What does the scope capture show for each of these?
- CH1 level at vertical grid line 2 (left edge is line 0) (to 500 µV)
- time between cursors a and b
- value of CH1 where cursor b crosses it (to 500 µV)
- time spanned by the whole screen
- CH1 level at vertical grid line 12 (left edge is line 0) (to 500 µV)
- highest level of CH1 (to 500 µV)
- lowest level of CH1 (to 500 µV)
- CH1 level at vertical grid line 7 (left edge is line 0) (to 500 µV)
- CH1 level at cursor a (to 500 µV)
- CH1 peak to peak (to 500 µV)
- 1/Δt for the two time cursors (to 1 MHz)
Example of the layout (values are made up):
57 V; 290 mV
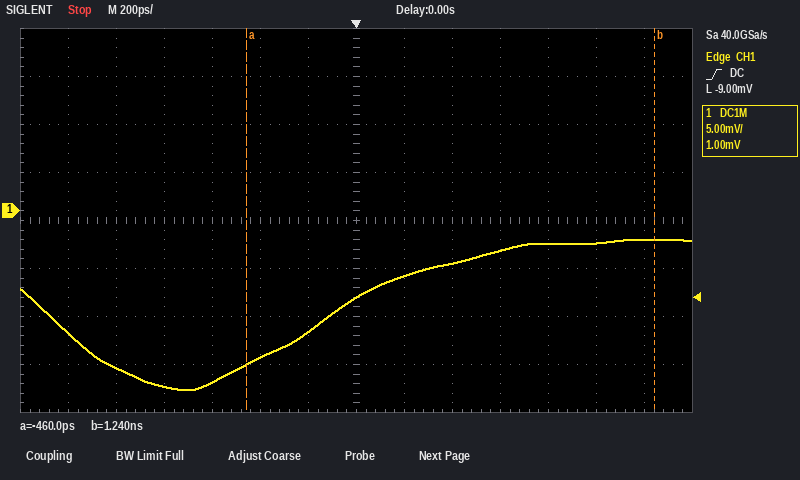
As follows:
-16.5 mV; 1.70 ns; -3.0 mV; 2.8 ns; -3.5 mV; -3.0 mV; -18.5 mV; -9.0 mV; -16.0 mV; 15.5 mV; 588 MHz
